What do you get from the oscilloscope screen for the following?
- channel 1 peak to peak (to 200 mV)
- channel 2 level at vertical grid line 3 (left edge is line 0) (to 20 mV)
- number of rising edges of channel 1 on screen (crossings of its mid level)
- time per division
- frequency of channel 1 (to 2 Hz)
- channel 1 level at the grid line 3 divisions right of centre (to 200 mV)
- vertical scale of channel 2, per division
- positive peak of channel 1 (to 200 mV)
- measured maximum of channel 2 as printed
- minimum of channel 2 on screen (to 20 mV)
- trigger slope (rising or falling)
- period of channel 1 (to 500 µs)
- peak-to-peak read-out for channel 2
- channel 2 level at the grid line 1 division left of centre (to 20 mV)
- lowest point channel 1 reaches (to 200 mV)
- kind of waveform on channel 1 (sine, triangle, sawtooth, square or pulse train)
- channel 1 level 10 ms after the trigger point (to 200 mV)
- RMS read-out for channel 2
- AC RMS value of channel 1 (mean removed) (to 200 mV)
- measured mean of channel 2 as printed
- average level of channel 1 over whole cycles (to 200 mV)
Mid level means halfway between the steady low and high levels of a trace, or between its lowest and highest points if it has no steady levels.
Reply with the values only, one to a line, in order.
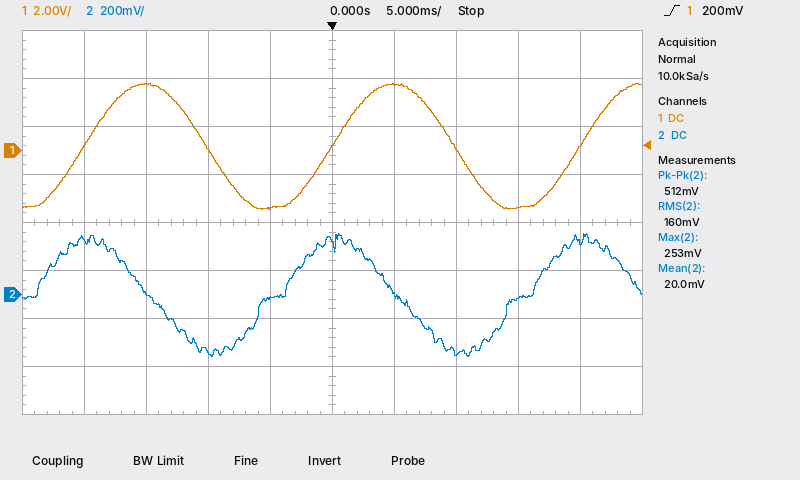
5.2 V
-240 mV
3
5 ms
50 Hz
-2.4 V
200 mV
2.8 V
253 mV
-260 mV
rising
20.0 ms
512 mV
-20 mV
-2.4 V
sine
0.0 V
160 mV
1.8 V
20.0 mV
200 mV
